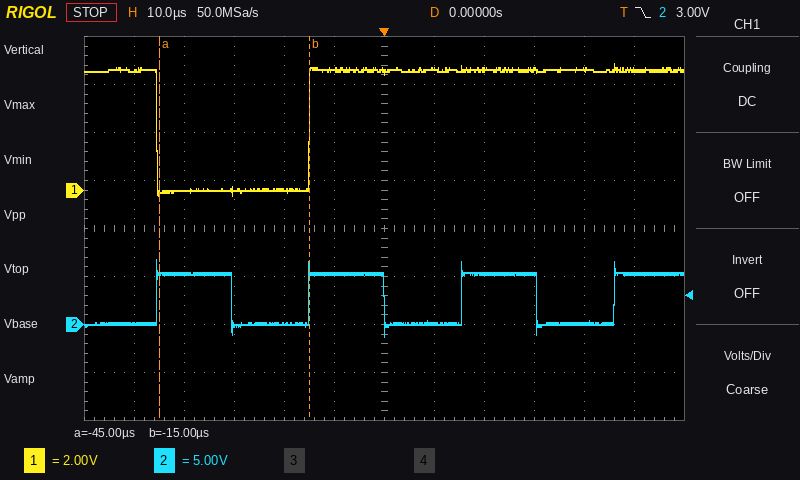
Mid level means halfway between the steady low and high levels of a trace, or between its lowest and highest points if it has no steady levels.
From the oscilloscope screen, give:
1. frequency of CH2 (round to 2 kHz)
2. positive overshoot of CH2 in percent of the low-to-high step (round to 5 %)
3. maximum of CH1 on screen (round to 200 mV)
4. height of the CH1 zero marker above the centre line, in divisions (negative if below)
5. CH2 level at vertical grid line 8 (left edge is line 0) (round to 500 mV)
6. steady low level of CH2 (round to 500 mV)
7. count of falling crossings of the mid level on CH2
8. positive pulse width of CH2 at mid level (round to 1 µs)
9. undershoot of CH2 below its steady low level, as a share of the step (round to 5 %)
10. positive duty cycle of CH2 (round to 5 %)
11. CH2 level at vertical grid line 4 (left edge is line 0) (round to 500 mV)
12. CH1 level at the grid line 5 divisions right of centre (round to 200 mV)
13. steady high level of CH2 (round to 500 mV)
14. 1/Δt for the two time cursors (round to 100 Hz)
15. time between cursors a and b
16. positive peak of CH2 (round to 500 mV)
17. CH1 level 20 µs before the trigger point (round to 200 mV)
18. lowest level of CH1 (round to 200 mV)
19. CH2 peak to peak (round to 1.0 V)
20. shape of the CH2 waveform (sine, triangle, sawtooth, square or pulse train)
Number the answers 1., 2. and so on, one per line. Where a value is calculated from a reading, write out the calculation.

1. 32 kHz
2. 30 %
3. 5.2 V
4. +0.8 div
5. 5.5 V
6. 0.0 V
7. 3
8. 15 µs
9. 25 %
10. 50 %
11. 0.0 V
12. 5.0 V
13. 5.5 V
14. 1 / 30 µs ≈ 33.3 kHz
15. -15 µs − (-45 µs) = 30 µs
16. 7.0 V
17. 0.0 V
18. -200 mV
19. 8.0 V
20. square
